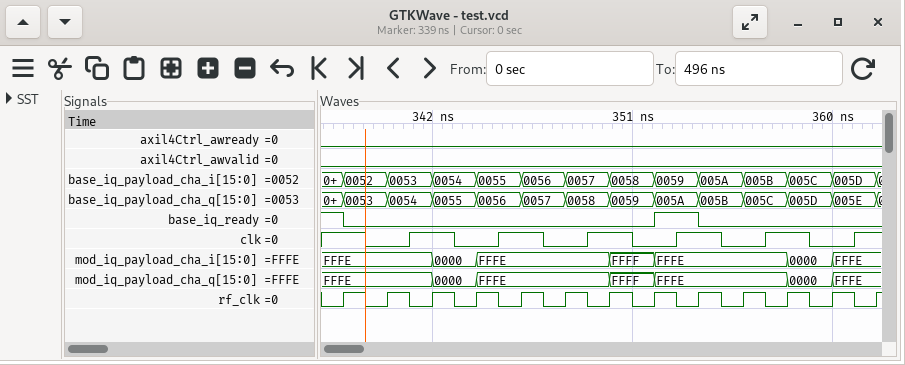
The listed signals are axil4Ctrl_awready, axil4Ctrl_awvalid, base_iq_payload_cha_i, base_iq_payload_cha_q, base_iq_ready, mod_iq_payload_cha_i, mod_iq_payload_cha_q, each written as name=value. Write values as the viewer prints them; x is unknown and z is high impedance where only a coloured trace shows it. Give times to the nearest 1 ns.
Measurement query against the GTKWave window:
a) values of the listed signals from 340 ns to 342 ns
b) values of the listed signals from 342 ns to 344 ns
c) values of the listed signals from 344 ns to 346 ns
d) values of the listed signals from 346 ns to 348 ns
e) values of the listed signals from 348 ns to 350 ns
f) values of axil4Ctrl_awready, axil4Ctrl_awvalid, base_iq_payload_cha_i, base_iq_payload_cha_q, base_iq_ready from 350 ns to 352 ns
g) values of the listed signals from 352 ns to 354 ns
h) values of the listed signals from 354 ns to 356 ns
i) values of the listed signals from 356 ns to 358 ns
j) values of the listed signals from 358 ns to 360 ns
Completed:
axil4Ctrl_awready=0, axil4Ctrl_awvalid=0, base_iq_payload_cha_i=0053, base_iq_payload_cha_q=0054, base_iq_ready=0, mod_iq_payload_cha_i=FFFE, mod_iq_payload_cha_q=FFFE
axil4Ctrl_awready=0, axil4Ctrl_awvalid=0, base_iq_payload_cha_i=0054, base_iq_payload_cha_q=0055, base_iq_ready=0, mod_iq_payload_cha_i=0000, mod_iq_payload_cha_q=0000
axil4Ctrl_awready=0, axil4Ctrl_awvalid=0, base_iq_payload_cha_i=0055, base_iq_payload_cha_q=0056, base_iq_ready=0, mod_iq_payload_cha_i=FFFE, mod_iq_payload_cha_q=FFFE
axil4Ctrl_awready=0, axil4Ctrl_awvalid=0, base_iq_payload_cha_i=0056, base_iq_payload_cha_q=0057, base_iq_ready=0, mod_iq_payload_cha_i=FFFE, mod_iq_payload_cha_q=FFFE
axil4Ctrl_awready=0, axil4Ctrl_awvalid=0, base_iq_payload_cha_i=0057, base_iq_payload_cha_q=0058, base_iq_ready=0, mod_iq_payload_cha_i=FFFE, mod_iq_payload_cha_q=FFFE
axil4Ctrl_awready=0, axil4Ctrl_awvalid=0, base_iq_payload_cha_i=0058, base_iq_payload_cha_q=0059, base_iq_ready=0
axil4Ctrl_awready=0, axil4Ctrl_awvalid=0, base_iq_payload_cha_i=0059, base_iq_payload_cha_q=005A, base_iq_ready=1, mod_iq_payload_cha_i=FFFE, mod_iq_payload_cha_q=FFFE
axil4Ctrl_awready=0, axil4Ctrl_awvalid=0, base_iq_payload_cha_i=005A, base_iq_payload_cha_q=005B, base_iq_ready=0, mod_iq_payload_cha_i=FFFE, mod_iq_payload_cha_q=FFFE
axil4Ctrl_awready=0, axil4Ctrl_awvalid=0, base_iq_payload_cha_i=005B, base_iq_payload_cha_q=005C, base_iq_ready=0, mod_iq_payload_cha_i=FFFE, mod_iq_payload_cha_q=FFFE
axil4Ctrl_awready=0, axil4Ctrl_awvalid=0, base_iq_payload_cha_i=005C, base_iq_payload_cha_q=005D, base_iq_ready=0, mod_iq_payload_cha_i=0000, mod_iq_payload_cha_q=0000
